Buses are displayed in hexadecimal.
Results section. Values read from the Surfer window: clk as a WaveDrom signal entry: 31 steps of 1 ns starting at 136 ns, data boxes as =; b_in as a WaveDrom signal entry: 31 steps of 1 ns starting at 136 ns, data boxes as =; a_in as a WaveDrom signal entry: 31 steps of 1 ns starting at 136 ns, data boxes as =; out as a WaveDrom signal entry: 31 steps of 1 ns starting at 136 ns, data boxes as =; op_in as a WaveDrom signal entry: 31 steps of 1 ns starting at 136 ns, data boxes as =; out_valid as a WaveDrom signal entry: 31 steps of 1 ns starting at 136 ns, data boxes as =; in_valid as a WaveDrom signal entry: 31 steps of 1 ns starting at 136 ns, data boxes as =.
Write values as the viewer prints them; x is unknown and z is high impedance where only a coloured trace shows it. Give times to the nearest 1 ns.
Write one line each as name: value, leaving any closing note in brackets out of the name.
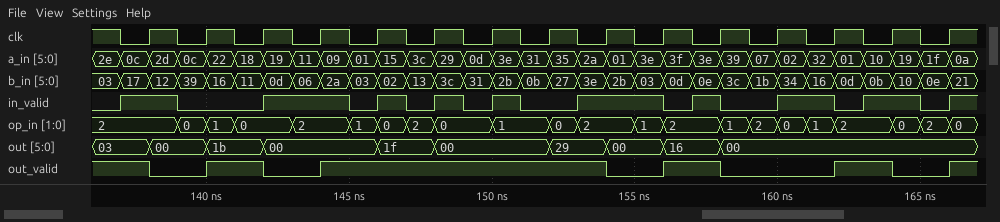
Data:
clk as a WaveDrom signal entry: 31 steps of 1 ns starting at 136 ns, data boxes as =: {name: 'clk', wave: '1010101010101010101010101010101'}
b_in as a WaveDrom signal entry: 31 steps of 1 ns starting at 136 ns, data boxes as =: {name: 'b_in', wave: '===============================', data: '03 17 12 39 16 11 0d 06 2a 03 02 13 3c 31 2b 0b 27 3e 2b 03 0d 0e 3c 1b 34 16 0d 0b 10 0e 21'}
a_in as a WaveDrom signal entry: 31 steps of 1 ns starting at 136 ns, data boxes as =: {name: 'a_in', wave: '===============================', data: '2e 0c 2d 0c 22 18 19 11 09 01 15 3c 29 0d 3e 31 35 2a 01 3e 3f 3e 39 07 02 32 01 10 19 1f 0a'}
out as a WaveDrom signal entry: 31 steps of 1 ns starting at 136 ns, data boxes as =: {name: 'out', wave: '=.=.=.=...=.=...=.=.=.=........', data: '03 00 1b 00 1f 00 29 00 16 00'}
op_in as a WaveDrom signal entry: 31 steps of 1 ns starting at 136 ns, data boxes as =: {name: 'op_in', wave: '=..===.=.====.=.==.==.=====.===', data: '2 0 1 0 2 1 0 2 0 1 0 2 1 2 1 2 0 1 2 0 2 0'}
out_valid as a WaveDrom signal entry: 31 steps of 1 ns starting at 136 ns, data boxes as =: {name: 'out_valid', wave: '1.0.1.0.1.........0.1.0...1.0.1'}
in_valid as a WaveDrom signal entry: 31 steps of 1 ns starting at 136 ns, data boxes as =: {name: 'in_valid', wave: '01.0..1..0101010.1..010.1.01.01'}
